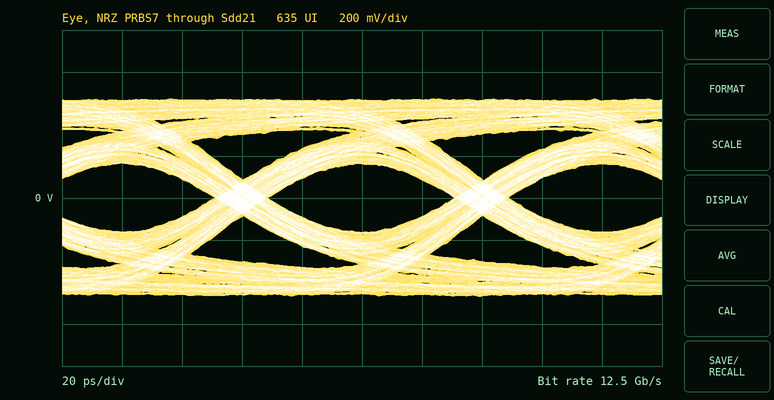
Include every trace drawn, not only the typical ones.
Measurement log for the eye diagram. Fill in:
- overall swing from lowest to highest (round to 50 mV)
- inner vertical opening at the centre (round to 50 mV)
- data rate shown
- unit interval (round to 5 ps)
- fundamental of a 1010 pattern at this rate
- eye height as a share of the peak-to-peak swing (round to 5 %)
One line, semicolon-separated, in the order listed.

950 mV; 350 mV; 12.5 Gb/s; 80 ps; 6.25 GHz; 35 %
